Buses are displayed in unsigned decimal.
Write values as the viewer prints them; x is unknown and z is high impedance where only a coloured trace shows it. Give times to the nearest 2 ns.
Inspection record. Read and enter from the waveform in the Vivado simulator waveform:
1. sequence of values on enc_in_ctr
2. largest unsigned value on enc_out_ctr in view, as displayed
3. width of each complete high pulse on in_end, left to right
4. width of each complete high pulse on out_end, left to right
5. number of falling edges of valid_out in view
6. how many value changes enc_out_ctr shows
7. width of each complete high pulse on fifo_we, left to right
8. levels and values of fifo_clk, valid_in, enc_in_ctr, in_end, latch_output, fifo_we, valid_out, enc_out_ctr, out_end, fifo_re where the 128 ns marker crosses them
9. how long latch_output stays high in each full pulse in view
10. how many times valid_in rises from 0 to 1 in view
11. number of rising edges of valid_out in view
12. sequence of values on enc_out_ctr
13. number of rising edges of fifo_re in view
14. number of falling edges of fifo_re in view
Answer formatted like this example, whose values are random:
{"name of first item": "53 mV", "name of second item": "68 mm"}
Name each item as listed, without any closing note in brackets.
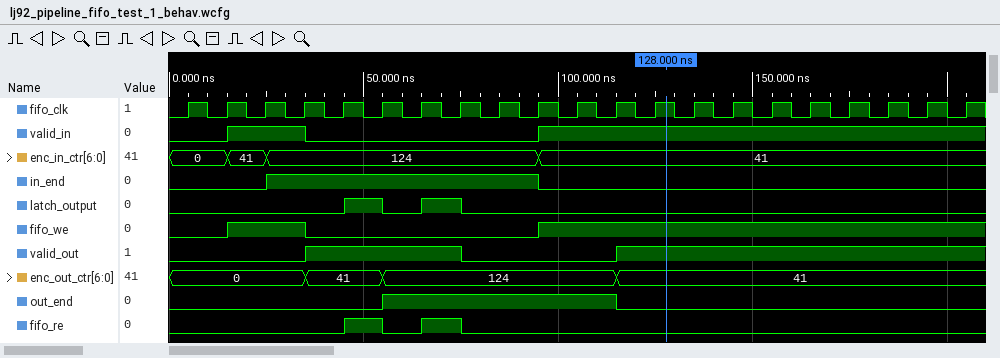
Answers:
{"sequence of values on enc_in_ctr": "0, 41, 124, 41", "largest unsigned value on enc_out_ctr in view, as displayed": "124", "width of each complete high pulse on in_end, left to right": "70 ns", "width of each complete high pulse on out_end, left to right": "60 ns", "number of falling edges of valid_out in view": "1", "how many value changes enc_out_ctr shows": "3", "width of each complete high pulse on fifo_we, left to right": "20 ns", "levels and values of fifo_clk, valid_in, enc_in_ctr, in_end, latch_output, fifo_we, valid_out, enc_out_ctr, out_end, fifo_re where the 128 ns marker crosses them": "fifo_clk=1, valid_in=1, enc_in_ctr=41, in_end=0, latch_output=0, fifo_we=1, valid_out=1, enc_out_ctr=41, out_end=0, fifo_re=0", "how long latch_output stays high in each full pulse in view": "10 ns, 10 ns", "how many times valid_in rises from 0 to 1 in view": "2", "number of rising edges of valid_out in view": "2", "sequence of values on enc_out_ctr": "0, 41, 124, 41", "number of rising edges of fifo_re in view": "2", "number of falling edges of fifo_re in view": "2"}
